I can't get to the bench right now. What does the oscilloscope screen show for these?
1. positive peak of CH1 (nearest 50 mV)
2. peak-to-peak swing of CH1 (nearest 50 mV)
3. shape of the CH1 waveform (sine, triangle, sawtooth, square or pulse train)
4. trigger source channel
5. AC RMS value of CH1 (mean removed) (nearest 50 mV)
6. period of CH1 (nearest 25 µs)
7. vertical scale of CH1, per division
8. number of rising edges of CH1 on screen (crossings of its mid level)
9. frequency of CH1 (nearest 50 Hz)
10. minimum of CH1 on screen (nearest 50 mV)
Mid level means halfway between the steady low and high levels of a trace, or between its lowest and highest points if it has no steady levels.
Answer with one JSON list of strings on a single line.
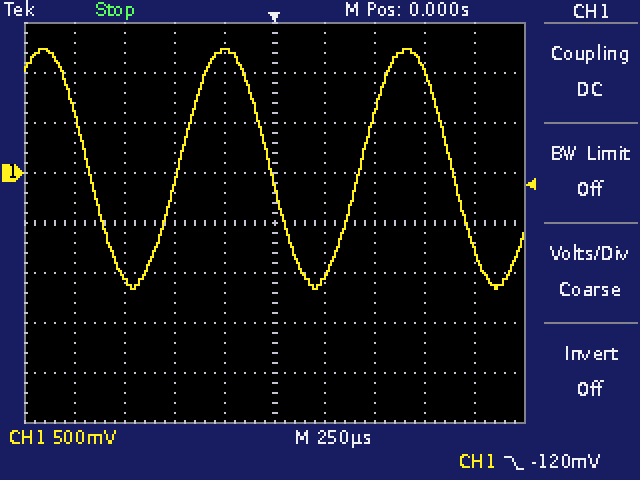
["1.25 V", "2.40 V", "sine", "CH1", "850 mV", "900 µs", "500 mV", "2", "1.10 kHz", "-1.15 V"]
